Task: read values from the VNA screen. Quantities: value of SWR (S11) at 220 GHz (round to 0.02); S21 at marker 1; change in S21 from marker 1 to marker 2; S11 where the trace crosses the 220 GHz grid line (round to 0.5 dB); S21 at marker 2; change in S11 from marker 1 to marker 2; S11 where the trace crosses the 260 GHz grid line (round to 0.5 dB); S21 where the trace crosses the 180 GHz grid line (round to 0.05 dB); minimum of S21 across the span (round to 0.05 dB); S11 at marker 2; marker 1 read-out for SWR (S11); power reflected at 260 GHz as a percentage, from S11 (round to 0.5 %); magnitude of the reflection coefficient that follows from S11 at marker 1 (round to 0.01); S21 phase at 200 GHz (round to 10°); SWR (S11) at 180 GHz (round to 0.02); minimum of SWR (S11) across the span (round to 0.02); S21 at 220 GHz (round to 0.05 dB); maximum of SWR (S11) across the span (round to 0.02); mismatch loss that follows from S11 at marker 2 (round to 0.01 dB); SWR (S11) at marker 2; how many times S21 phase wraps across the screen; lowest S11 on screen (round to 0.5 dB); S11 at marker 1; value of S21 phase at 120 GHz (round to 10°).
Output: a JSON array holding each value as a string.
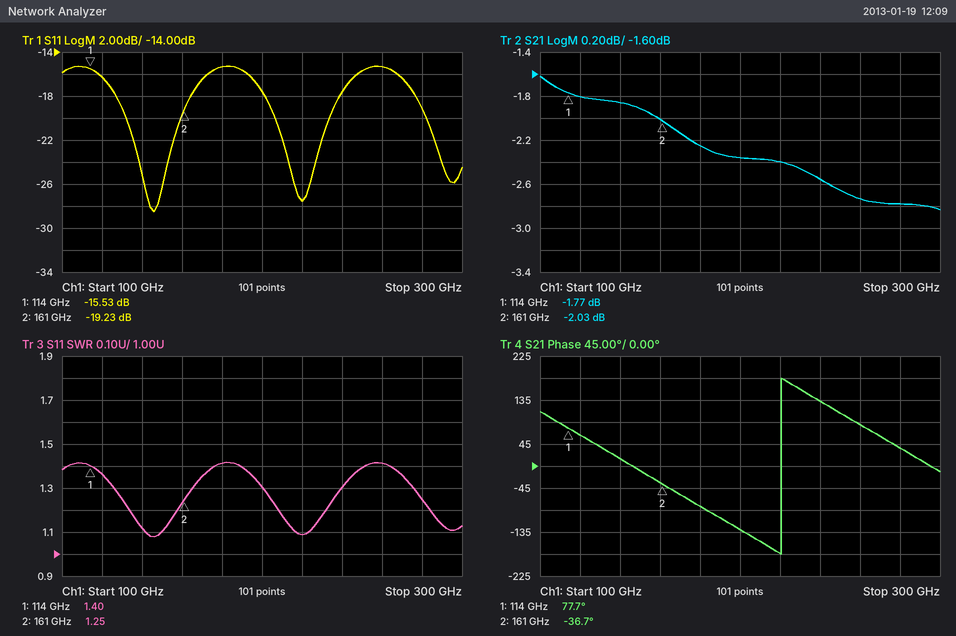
["1.08", "-1.77 dB", "-0.26 dB", "-27.5 dB", "-2.03 dB", "-3.70 dB", "-15.5 dB", "-2.25 dB", "-2.85 dB", "-19.23 dB", "1.40", "3.0 %", "0.17", "-130°", "1.42", "1.08", "-2.40 dB", "1.42", "0.05 dB", "1.25", "1", "-28.5 dB", "-15.53 dB", "60°"]
